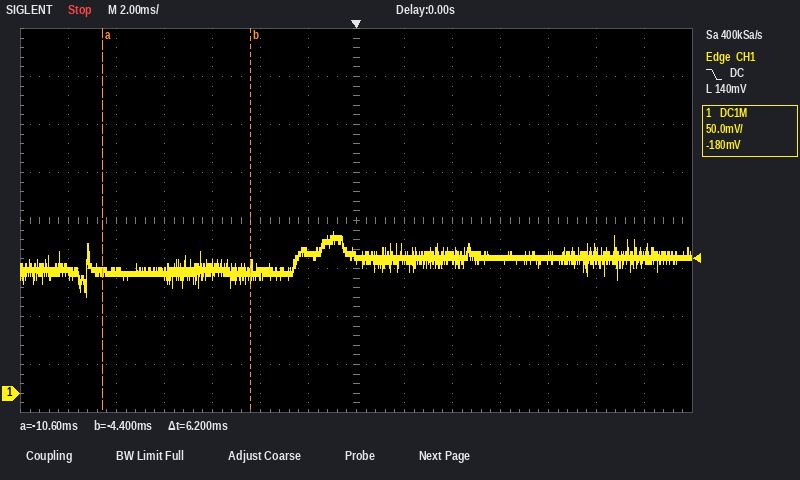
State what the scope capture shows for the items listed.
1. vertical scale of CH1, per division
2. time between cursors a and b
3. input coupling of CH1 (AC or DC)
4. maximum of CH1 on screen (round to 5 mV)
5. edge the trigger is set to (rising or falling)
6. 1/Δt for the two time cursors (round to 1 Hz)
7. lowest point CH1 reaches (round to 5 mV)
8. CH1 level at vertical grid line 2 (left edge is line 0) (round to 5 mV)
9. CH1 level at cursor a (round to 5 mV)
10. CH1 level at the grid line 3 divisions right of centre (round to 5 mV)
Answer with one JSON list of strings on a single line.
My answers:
["50 mV", "6.2 ms", "DC", "170 mV", "falling", "161 Hz", "100 mV", "125 mV", "125 mV", "140 mV"]
